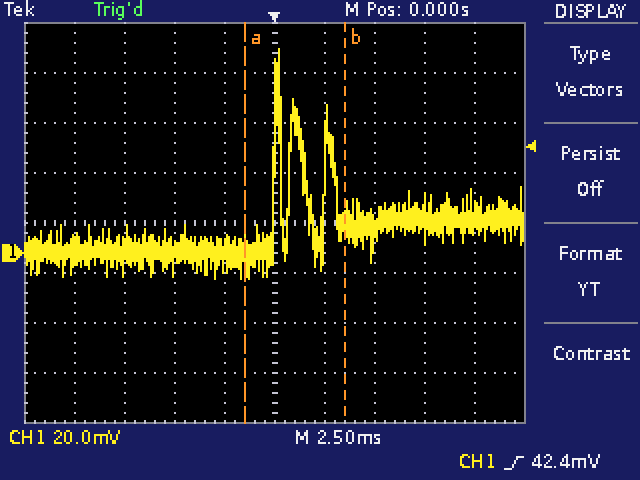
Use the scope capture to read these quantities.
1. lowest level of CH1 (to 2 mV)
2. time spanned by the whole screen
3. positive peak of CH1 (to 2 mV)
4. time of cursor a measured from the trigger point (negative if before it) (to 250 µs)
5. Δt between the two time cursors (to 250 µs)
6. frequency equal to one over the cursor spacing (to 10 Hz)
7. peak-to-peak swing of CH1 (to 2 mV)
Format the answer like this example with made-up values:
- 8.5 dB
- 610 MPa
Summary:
- -10 mV
- 25 ms
- 82 mV
- -1.50 ms
- 5.00 ms
- 200 Hz
- 92 mV
